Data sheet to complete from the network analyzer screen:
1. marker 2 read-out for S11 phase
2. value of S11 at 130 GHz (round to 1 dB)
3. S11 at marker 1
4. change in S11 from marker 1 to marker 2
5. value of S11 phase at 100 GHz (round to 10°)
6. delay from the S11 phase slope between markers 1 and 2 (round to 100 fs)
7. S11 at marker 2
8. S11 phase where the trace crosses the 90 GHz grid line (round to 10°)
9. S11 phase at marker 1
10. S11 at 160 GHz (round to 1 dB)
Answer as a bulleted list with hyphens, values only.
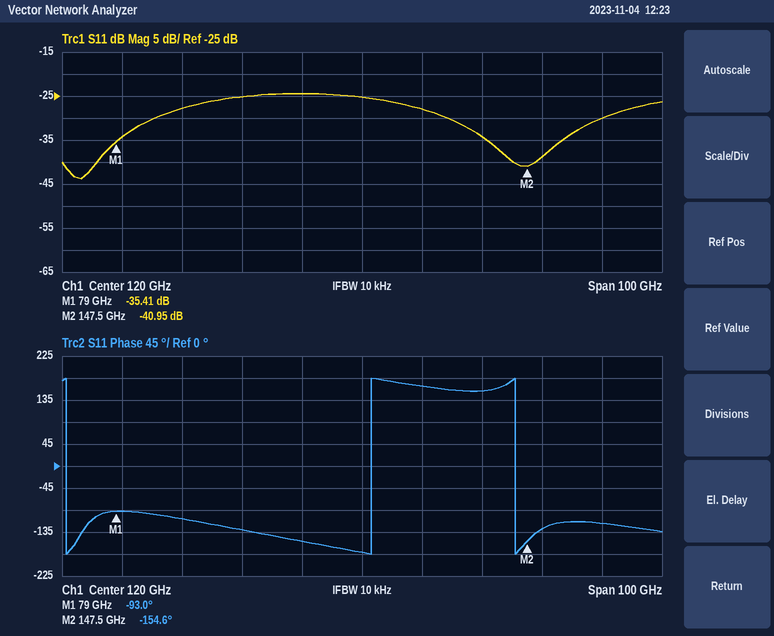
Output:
- -154.6°
- -28 dB
- -35.41 dB
- -5.54 dB
- -130°
- 2.5 ps
- -40.95 dB
- -110°
- -93.0°
- -30 dB
